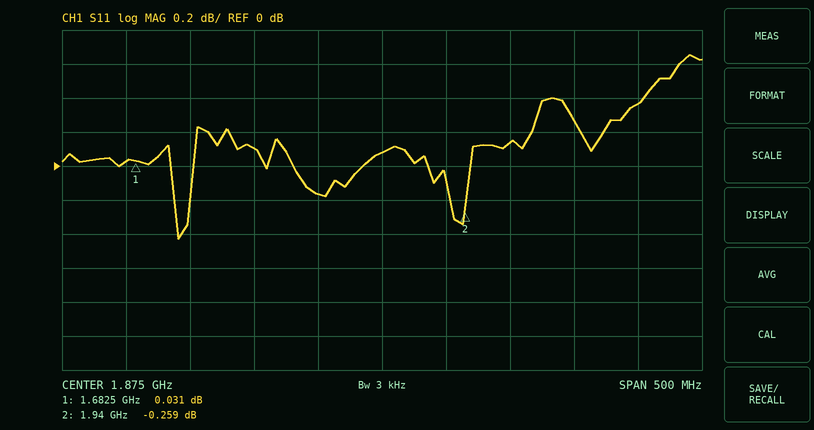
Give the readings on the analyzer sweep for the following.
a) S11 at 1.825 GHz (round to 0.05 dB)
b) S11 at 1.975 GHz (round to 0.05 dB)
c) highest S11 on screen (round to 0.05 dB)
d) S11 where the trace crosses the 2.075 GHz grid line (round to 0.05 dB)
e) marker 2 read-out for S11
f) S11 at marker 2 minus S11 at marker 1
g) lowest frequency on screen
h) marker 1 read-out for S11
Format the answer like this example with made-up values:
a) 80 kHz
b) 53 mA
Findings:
a) -0.15 dB
b) 0.15 dB
c) 0.65 dB
d) 0.35 dB
e) -0.259 dB
f) -0.290 dB
g) 1.625 GHz
h) 0.031 dB
